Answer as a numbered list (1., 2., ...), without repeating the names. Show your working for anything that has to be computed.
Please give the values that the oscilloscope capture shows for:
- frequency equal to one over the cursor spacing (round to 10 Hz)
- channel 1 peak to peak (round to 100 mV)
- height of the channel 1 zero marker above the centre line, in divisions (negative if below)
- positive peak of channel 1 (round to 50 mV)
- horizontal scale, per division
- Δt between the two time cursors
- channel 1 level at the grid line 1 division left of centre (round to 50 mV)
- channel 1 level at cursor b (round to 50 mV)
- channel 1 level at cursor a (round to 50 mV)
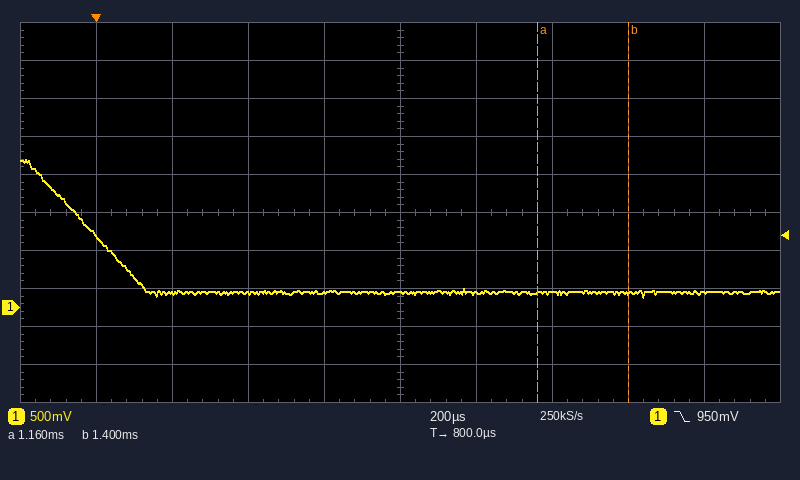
1. 1 / 240 µs ≈ 4.17 kHz
2. 1.80 V
3. -2.5 div
4. 1.95 V
5. 200 µs
6. 1.4 ms − (1.16 ms) = 240 µs
7. 200 mV
8. 200 mV
9. 200 mV
